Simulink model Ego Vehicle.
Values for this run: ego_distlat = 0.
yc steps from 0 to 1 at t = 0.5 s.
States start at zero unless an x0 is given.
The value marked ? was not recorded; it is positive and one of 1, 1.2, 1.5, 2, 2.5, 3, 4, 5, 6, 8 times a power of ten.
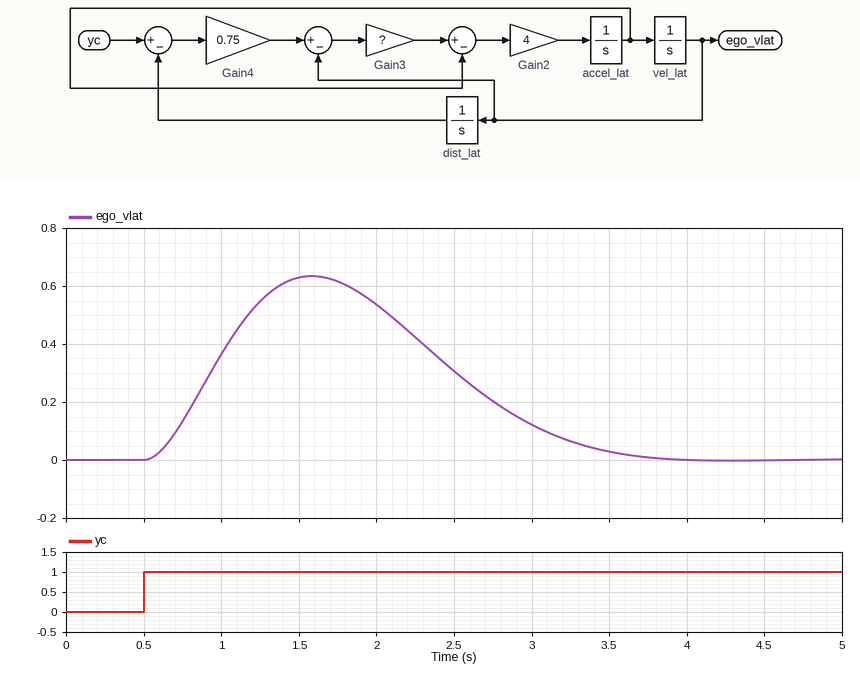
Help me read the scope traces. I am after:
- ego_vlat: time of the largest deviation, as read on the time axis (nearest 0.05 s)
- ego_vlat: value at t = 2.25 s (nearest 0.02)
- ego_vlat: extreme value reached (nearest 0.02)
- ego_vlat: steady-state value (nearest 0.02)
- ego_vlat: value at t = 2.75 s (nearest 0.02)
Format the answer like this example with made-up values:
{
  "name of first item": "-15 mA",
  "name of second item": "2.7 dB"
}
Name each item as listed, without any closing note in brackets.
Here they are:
{
  "ego_vlat: time of the largest deviation, as read on the time axis": "1.60 s",
  "ego_vlat: value at t = 2.25 s": "0.42",
  "ego_vlat: extreme value reached": "0.64",
  "ego_vlat: steady-state value": "0.00",
  "ego_vlat: value at t = 2.75 s": "0.20"
}
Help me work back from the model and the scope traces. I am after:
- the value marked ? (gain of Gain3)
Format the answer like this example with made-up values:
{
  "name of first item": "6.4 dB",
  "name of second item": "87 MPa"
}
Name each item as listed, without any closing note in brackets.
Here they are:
{
  "the value marked ?": "2"
}
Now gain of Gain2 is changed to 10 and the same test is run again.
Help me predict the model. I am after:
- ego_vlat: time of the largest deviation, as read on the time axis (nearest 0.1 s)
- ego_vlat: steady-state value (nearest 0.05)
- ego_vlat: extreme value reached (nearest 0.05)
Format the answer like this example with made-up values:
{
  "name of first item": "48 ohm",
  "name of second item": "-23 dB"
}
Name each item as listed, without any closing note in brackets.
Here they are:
{
  "ego_vlat: time of the largest deviation, as read on the time axis": "1.4 s",
  "ego_vlat: steady-state value": "0.00",
  "ego_vlat: extreme value reached": "0.55"
}
